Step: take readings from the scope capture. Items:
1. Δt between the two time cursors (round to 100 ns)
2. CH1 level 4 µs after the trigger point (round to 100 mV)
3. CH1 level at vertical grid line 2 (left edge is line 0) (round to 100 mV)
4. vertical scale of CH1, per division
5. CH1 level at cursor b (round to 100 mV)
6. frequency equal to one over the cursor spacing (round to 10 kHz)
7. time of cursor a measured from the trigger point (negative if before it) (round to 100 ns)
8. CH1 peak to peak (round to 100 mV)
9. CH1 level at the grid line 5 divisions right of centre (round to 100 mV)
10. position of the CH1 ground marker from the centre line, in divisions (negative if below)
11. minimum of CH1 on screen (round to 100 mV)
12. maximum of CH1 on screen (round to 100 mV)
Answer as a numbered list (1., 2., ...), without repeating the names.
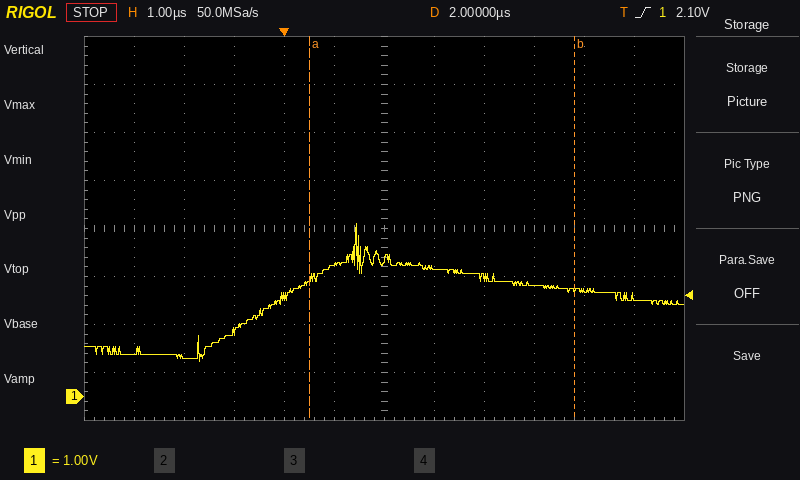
1. 5.3 µs
2. 2.5 V
3. 800 mV
4. 1 V
5. 2.2 V
6. 190 kHz
7. +500 ns
8. 2.9 V
9. 2.1 V
10. -3.5 div
11. 700 mV
12. 3.6 V
